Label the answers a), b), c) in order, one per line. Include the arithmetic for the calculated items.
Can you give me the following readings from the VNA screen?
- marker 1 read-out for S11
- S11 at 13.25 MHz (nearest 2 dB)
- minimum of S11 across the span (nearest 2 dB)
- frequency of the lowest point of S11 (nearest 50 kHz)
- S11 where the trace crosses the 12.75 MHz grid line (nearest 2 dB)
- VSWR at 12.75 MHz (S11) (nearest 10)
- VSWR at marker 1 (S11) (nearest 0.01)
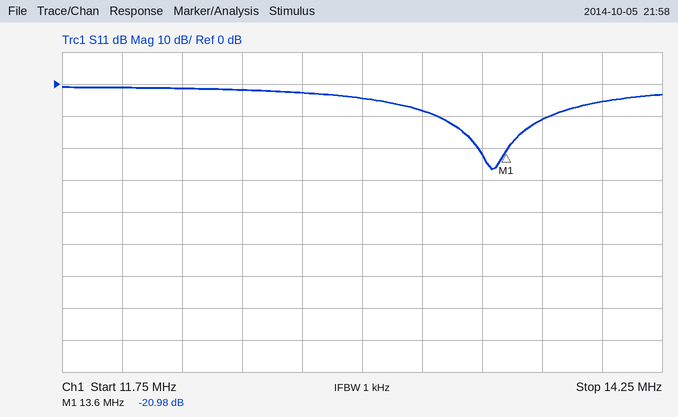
a) -20.98 dB
b) -8 dB
c) -26 dB
d) 13.55 MHz
e) -2 dB
f) |Γ| = 10^(-2/20) = 0.7943; VSWR = (1 + 0.7943)/(1 − 0.7943) ≈ 8.72, so 10 to the nearest 10
g) (1 + 0.0893)/(1 − 0.0893) ≈ 1.20
